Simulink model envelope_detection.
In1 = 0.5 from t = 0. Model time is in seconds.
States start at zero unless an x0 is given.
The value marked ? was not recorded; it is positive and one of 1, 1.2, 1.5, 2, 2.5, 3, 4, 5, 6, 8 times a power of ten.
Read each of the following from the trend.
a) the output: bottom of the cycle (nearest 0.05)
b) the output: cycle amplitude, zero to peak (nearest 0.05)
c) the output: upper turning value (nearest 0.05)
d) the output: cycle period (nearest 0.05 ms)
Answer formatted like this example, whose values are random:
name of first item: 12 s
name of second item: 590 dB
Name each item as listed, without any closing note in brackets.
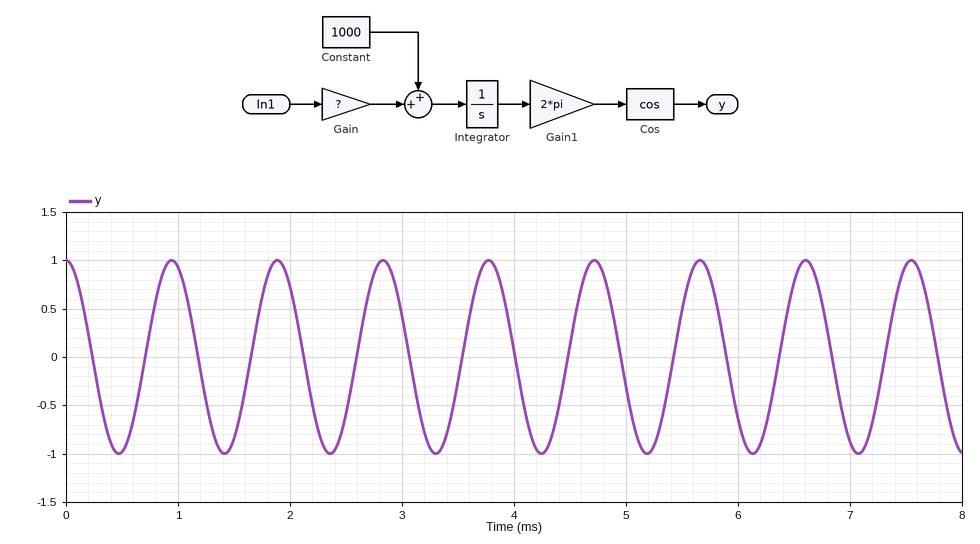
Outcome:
the output: bottom of the cycle: -1.00
the output: cycle amplitude, zero to peak: 1.00
the output: upper turning value: 1.00
the output: cycle period: 0.95 ms
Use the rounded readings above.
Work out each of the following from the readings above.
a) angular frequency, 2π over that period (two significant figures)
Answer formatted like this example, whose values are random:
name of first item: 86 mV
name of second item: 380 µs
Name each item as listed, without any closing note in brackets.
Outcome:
angular frequency, 2π over that period: 6.6 rad/ms
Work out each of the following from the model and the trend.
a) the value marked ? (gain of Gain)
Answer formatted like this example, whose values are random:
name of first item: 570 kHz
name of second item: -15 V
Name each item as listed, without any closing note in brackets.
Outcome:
the value marked ?: 120
